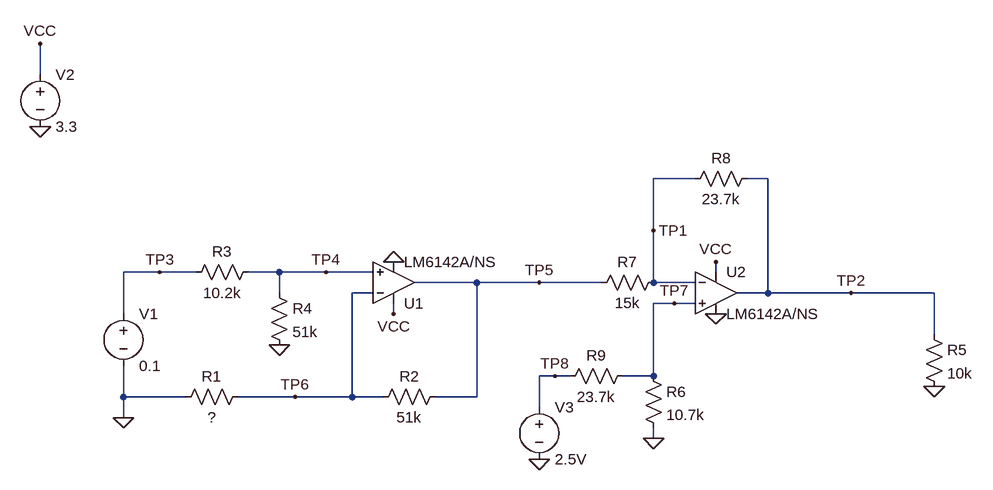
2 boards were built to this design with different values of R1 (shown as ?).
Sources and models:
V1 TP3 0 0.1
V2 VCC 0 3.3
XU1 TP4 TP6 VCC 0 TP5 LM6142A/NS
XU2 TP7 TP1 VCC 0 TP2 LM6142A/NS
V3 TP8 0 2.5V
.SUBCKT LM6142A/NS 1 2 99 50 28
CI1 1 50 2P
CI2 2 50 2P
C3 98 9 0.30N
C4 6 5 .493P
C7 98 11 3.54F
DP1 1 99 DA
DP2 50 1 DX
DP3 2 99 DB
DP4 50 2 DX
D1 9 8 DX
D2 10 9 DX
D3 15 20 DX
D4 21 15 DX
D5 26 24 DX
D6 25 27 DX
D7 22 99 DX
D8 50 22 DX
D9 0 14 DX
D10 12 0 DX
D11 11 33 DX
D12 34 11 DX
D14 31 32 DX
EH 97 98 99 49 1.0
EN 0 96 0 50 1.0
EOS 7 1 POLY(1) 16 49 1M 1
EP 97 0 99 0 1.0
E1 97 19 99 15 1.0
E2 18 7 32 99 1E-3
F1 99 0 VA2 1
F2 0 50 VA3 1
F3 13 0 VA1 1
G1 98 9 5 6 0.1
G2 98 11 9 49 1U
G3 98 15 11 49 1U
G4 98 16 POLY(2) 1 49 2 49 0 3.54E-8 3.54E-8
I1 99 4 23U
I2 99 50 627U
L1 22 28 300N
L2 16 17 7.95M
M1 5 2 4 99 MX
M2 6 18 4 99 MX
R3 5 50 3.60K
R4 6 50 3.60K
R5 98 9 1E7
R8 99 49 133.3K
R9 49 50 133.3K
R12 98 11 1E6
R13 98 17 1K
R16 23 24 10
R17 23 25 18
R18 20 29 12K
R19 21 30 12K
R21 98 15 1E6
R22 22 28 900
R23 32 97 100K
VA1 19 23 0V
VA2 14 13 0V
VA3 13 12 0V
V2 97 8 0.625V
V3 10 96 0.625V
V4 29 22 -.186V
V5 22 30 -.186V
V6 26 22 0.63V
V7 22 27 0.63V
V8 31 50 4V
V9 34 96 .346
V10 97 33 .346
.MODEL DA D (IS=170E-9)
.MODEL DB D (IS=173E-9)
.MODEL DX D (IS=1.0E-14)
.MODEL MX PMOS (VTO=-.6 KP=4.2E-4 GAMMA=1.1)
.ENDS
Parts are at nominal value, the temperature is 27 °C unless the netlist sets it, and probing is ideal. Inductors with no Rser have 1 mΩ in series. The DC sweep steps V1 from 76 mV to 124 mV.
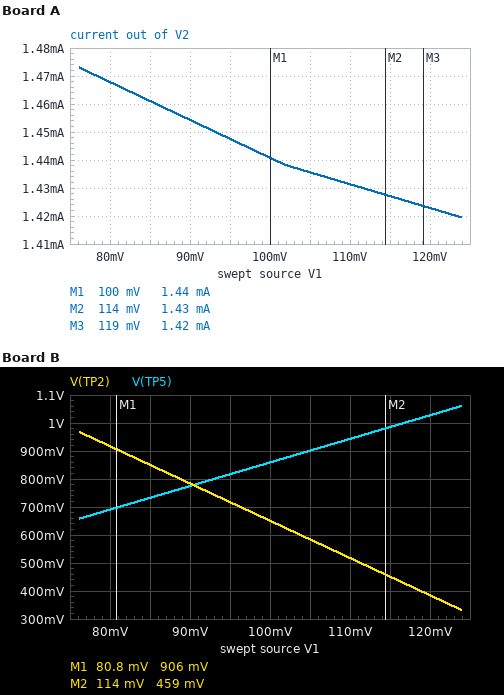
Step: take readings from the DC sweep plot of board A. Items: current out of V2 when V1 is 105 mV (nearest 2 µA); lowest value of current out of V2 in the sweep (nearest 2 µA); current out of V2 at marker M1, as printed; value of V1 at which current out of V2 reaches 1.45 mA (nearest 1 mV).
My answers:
1.436 mA
1.420 mA
1.44 mA
93 mV
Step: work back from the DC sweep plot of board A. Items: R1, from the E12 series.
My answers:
8.2 kΩ
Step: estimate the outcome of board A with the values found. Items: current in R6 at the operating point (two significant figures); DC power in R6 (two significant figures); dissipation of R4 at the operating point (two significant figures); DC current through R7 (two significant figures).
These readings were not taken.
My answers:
73 µA
57 µW
140 nW
11 µA
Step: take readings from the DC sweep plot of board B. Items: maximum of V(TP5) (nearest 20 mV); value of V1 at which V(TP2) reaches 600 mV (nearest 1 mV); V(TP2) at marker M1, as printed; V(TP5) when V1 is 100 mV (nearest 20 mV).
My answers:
1.06 V
104 mV
906 mV
860 mV
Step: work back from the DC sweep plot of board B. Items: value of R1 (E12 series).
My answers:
5.6 kΩ
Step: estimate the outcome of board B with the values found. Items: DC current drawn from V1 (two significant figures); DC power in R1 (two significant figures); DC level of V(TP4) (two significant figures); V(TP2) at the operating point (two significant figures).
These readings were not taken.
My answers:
1.5 µA
1.3 µW
85 mV
650 mV
